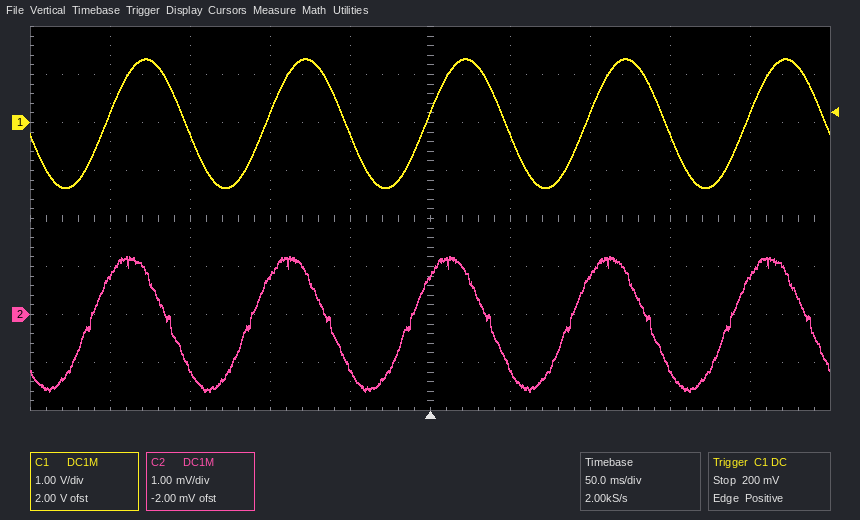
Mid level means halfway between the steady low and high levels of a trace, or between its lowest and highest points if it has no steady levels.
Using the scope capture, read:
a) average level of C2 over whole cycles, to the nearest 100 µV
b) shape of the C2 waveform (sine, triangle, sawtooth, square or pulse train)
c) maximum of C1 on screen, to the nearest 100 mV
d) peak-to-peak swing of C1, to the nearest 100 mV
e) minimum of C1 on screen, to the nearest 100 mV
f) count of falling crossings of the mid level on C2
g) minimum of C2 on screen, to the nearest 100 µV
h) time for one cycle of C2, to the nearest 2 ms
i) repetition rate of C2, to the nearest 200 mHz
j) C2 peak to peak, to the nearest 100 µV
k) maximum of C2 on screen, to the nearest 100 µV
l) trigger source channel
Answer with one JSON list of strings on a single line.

["-200 µV", "sine", "1.3 V", "2.7 V", "-1.4 V", "5", "-1.6 mV", "100 ms", "10.0 Hz", "2.8 mV", "1.2 mV", "C1"]
